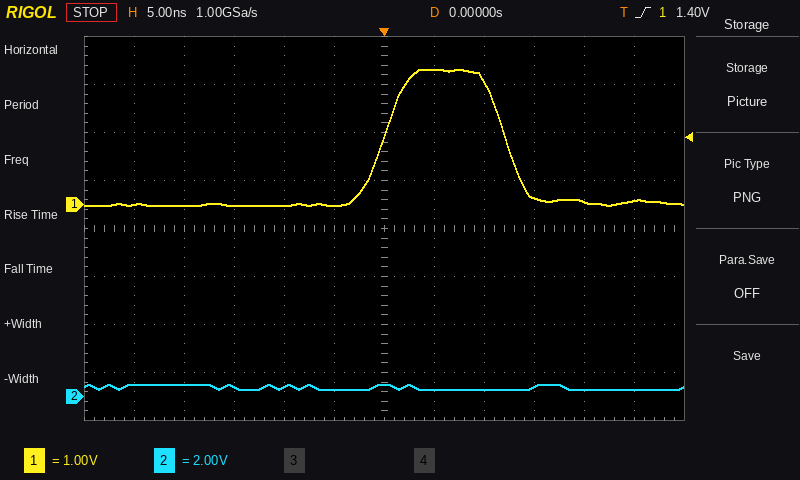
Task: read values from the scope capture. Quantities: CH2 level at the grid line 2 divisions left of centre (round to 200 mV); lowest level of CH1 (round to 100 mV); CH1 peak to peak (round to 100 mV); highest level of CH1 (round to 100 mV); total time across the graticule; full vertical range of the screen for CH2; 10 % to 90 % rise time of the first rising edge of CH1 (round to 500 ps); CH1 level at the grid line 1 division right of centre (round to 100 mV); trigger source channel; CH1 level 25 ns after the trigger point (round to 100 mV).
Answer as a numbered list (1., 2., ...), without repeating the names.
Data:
1. 400 mV
2. 0.0 V
3. 2.8 V
4. 2.8 V
5. 60 ns
6. 16 V
7. 4.5 ns
8. 2.8 V
9. CH1
10. 100 mV
